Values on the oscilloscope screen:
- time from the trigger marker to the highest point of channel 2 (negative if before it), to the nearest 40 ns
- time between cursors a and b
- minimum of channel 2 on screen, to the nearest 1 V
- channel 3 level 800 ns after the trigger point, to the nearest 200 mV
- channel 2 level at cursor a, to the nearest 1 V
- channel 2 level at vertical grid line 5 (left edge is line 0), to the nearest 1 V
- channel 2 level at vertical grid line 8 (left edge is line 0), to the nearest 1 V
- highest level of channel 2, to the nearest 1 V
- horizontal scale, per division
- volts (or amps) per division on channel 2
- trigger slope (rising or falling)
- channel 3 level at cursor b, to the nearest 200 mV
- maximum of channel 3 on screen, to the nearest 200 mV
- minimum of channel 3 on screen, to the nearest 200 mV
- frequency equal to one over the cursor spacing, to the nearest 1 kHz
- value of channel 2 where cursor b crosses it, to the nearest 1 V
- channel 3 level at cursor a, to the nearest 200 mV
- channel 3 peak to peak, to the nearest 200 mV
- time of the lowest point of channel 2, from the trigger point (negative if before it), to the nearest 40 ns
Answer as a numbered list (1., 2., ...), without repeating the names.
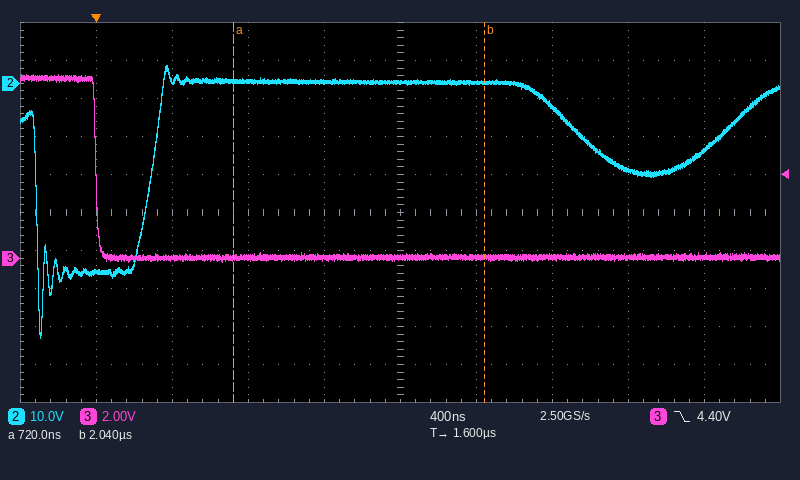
1. +360 ns
2. 1.32 µs
3. -67 V
4. 0.0 V
5. 1 V
6. 0 V
7. -23 V
8. 5 V
9. 400 ns
10. 10 V
11. falling
12. 0.0 V
13. 9.6 V
14. -200 mV
15. 758 kHz
16. 0 V
17. 0.0 V
18. 9.8 V
19. -280 ns
